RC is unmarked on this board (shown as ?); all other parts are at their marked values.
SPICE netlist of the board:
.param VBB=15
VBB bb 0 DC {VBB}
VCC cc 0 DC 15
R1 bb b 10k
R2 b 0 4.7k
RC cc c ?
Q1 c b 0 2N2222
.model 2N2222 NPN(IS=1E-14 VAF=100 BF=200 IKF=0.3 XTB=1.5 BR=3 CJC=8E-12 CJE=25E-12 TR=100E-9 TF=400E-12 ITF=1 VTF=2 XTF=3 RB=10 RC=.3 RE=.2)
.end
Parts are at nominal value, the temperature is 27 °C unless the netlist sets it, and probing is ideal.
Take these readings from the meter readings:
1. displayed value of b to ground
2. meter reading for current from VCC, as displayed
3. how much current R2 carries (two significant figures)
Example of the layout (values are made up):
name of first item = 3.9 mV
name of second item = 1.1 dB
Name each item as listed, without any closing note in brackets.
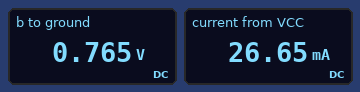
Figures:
displayed value of b to ground = 0.765 V
meter reading for current from VCC, as displayed = 26.65 mA
how much current R2 carries = 160 µA
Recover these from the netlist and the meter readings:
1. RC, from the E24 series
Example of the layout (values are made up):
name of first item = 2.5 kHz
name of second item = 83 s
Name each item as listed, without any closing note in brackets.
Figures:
RC, from the E24 series = 560 Ω
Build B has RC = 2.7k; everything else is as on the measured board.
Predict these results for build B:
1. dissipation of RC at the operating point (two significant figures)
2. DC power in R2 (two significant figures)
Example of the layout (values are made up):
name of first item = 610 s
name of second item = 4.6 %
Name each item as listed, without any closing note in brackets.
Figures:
dissipation of RC at the operating point = 83 mW
DC power in R2 = 110 µW
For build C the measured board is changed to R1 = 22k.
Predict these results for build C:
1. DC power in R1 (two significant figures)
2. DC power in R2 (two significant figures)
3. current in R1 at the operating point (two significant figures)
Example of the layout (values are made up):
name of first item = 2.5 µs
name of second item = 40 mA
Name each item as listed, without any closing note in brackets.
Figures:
DC power in R1 = 9.2 mW
DC power in R2 = 120 µW
current in R1 at the operating point = 650 µA
